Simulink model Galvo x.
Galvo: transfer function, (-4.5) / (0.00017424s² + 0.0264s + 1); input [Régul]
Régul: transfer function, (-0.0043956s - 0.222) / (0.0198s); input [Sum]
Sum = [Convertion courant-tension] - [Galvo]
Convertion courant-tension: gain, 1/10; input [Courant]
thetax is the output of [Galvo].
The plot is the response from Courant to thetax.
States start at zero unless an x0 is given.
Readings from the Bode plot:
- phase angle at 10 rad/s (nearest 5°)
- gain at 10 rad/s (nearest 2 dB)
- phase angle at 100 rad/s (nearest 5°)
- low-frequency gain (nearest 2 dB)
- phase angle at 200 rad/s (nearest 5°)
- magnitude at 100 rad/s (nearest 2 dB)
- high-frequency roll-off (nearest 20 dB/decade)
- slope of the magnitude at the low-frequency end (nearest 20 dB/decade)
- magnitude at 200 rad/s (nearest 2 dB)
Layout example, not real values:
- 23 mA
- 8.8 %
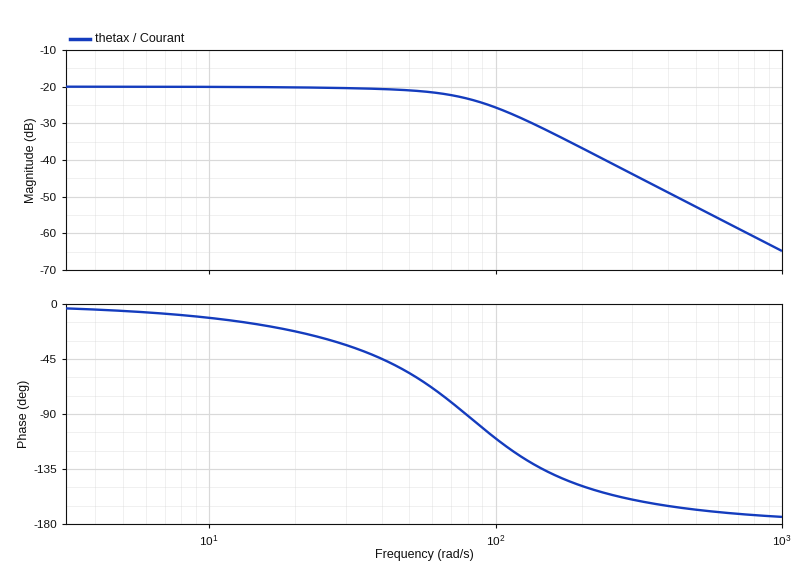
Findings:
- -10°
- -20 dB
- -110°
- -20 dB
- -150°
- -26 dB
- -40 dB/decade
- 0 dB/decade
- -36 dB
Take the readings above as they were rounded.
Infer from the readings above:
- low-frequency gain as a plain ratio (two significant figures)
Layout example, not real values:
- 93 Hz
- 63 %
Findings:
- 0.10
